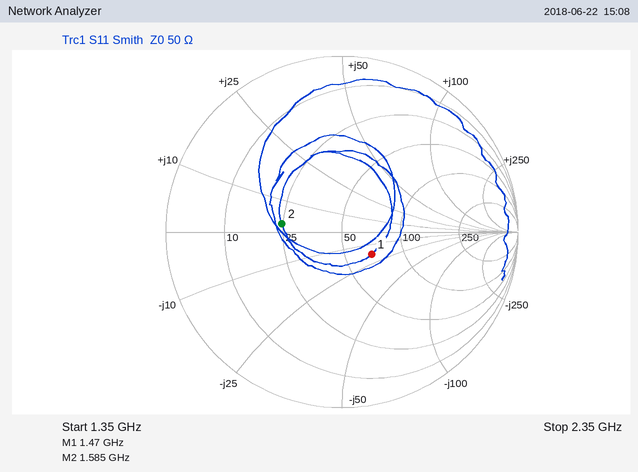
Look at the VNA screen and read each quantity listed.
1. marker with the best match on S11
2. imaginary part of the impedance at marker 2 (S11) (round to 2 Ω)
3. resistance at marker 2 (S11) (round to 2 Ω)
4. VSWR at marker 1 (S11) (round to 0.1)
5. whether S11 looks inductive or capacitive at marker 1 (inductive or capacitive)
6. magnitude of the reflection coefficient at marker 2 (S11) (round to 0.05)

marker 1
+2 Ω
24 Ω
1.5
capacitive
0.35
